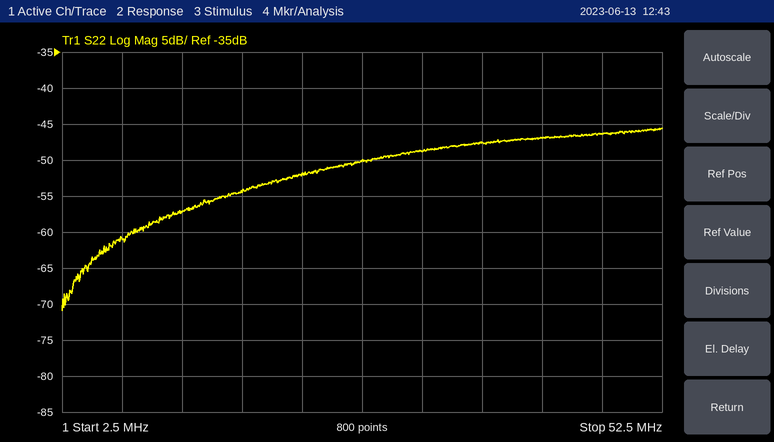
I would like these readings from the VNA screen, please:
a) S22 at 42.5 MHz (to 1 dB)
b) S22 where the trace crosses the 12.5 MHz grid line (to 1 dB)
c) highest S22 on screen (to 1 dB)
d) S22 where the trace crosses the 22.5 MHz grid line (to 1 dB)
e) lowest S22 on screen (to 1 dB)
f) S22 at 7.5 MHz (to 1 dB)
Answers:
-47 dB
-57 dB
-46 dB
-52 dB
-71 dB
-61 dB
